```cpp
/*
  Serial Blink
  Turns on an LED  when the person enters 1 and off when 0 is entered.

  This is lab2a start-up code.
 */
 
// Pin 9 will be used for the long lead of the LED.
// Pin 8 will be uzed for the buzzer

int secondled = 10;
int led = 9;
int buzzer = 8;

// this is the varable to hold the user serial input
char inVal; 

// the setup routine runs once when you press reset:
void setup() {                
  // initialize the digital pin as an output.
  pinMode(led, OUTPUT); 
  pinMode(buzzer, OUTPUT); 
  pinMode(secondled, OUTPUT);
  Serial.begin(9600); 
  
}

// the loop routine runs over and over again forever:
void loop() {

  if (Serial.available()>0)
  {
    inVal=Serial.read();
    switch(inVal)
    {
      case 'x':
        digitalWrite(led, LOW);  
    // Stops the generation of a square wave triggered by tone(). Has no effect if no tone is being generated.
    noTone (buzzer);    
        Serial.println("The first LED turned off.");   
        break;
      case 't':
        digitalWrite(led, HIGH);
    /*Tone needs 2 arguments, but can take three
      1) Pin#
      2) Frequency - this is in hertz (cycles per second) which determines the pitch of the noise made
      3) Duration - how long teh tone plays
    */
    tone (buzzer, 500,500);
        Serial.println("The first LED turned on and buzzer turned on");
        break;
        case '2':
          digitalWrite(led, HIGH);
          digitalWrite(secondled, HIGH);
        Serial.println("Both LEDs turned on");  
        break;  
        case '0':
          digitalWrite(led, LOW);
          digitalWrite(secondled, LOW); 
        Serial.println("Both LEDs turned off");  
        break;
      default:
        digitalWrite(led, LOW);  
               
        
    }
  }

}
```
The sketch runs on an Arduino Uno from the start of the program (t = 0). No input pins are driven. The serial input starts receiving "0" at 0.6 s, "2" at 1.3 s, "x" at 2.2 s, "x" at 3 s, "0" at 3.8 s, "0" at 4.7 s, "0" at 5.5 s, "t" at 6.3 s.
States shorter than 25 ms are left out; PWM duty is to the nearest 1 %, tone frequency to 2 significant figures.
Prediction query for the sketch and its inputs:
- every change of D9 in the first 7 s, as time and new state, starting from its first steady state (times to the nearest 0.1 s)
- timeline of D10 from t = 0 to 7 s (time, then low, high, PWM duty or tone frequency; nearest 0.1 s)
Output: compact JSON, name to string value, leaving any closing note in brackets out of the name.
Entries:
{"every change of D9 in the first 7 s, as time and new state, starting from its first steady state": "0 s low; 1.3 s high; 2.2 s low; 6.3 s high", "timeline of D10 from t = 0 to 7 s": "0 s low; 1.3 s high; 3.8 s low"}
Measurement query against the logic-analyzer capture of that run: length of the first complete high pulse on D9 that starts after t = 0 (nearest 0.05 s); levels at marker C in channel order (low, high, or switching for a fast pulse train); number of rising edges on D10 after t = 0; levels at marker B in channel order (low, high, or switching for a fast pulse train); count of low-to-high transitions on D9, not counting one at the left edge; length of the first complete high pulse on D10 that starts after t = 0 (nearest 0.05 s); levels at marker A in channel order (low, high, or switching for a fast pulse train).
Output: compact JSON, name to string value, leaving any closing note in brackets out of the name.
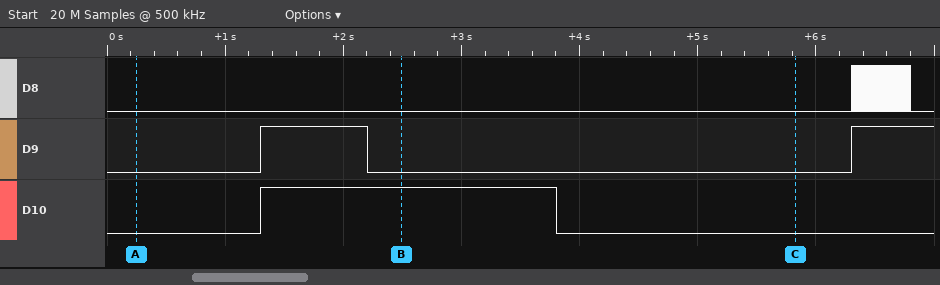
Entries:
{"length of the first complete high pulse on D9 that starts after t = 0": "0.90 s", "levels at marker C in channel order": "D8 low, D9 low, D10 low", "number of rising edges on D10 after t = 0": "1", "levels at marker B in channel order": "D8 low, D9 low, D10 high", "count of low-to-high transitions on D9, not counting one at the left edge": "2", "length of the first complete high pulse on D10 that starts after t = 0": "2.50 s", "levels at marker A in channel order": "D8 low, D9 low, D10 low"}
